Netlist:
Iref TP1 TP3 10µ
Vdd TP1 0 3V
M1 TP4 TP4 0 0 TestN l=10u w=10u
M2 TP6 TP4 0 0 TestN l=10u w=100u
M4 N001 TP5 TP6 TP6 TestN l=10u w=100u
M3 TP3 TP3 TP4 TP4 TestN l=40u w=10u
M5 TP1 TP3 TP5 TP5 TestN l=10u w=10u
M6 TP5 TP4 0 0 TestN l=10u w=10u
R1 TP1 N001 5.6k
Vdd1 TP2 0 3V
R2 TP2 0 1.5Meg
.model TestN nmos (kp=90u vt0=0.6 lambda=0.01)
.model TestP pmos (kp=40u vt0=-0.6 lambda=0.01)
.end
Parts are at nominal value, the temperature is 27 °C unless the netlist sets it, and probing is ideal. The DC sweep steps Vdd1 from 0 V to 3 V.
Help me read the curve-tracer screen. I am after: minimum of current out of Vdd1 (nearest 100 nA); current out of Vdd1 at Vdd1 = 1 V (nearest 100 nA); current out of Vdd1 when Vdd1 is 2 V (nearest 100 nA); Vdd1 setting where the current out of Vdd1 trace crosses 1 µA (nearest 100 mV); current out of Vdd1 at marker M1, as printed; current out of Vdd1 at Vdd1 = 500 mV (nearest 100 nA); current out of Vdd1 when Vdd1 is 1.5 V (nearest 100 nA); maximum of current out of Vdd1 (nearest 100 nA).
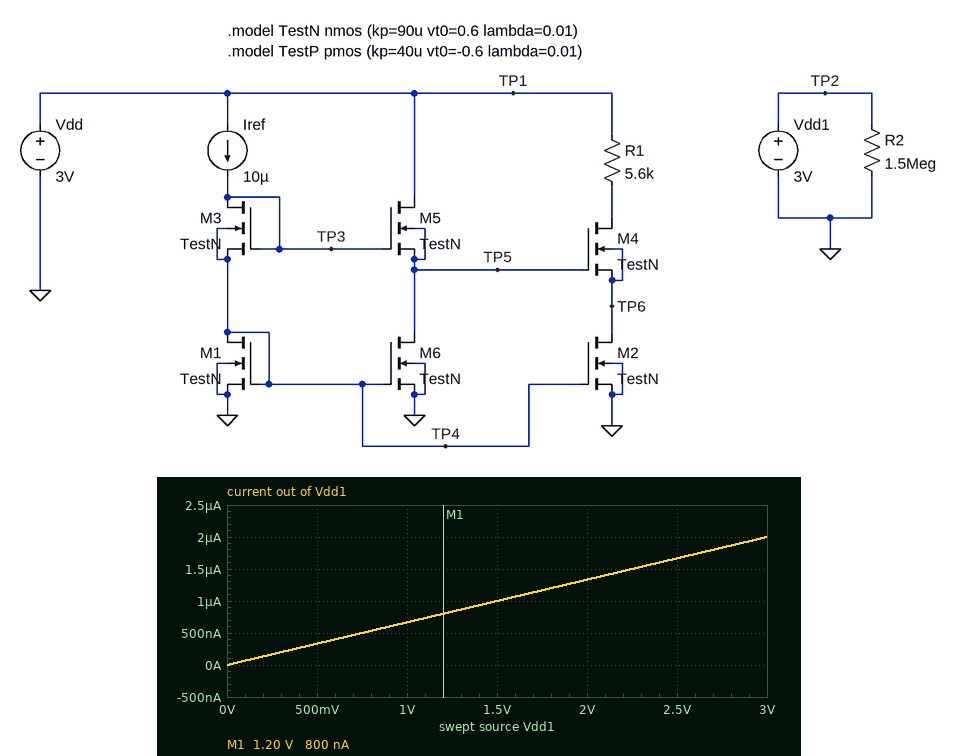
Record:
0 A
700 nA
1.3 µA
1.5 V
800 nA
300 nA
1.0 µA
2.0 µA
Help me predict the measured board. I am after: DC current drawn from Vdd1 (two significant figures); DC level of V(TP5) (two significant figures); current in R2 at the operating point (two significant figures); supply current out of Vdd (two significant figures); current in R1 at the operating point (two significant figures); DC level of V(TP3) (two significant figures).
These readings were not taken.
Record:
2.0 µA
1.5 V
2.0 µA
120 µA
99 µA
2.6 V
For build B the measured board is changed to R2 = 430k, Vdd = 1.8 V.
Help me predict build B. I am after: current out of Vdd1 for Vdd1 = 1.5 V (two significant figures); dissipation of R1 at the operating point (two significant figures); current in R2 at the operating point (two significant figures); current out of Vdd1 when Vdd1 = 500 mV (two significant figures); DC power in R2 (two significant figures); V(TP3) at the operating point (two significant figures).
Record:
3.5 µA
54 µW
7.0 µA
1.2 µA
21 µW
2.6 V
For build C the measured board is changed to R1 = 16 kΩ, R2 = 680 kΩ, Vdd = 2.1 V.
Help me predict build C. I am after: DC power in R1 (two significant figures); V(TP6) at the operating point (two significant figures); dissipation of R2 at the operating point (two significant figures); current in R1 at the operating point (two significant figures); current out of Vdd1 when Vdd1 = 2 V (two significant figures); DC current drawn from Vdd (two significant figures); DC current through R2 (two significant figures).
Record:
140 µW
360 mV
13 µW
94 µA
2.9 µA
110 µA
4.4 µA
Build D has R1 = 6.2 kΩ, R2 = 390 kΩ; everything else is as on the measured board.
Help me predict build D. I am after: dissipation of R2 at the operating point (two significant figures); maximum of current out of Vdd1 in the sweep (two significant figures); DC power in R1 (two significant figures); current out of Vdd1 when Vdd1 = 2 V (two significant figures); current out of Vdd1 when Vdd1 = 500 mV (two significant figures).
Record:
23 µW
7.7 µA
61 µW
5.1 µA
1.3 µA
